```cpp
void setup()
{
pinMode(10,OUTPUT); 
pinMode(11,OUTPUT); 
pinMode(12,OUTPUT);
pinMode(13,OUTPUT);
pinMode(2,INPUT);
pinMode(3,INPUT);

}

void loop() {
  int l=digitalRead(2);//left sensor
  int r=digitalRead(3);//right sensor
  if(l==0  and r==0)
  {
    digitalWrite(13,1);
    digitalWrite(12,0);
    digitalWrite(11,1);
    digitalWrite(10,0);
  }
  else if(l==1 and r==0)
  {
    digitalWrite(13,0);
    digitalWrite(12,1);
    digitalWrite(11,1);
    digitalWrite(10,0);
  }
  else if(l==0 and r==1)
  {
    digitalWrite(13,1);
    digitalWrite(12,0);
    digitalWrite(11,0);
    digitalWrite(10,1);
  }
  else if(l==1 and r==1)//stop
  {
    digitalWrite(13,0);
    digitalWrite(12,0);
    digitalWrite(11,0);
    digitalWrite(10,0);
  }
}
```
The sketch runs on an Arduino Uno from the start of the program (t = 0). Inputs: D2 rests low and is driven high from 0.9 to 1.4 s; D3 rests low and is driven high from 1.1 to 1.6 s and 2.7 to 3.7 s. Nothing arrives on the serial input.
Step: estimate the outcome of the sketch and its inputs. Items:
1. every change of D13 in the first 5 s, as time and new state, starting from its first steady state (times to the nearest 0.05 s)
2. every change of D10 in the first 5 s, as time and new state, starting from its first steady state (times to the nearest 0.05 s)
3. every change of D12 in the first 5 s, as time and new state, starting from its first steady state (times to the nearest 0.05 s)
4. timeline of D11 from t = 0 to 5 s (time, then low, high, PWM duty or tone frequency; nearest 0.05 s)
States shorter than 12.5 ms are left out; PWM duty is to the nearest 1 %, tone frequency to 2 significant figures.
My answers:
0 s high; 0.9 s low; 1.4 s high
0 s low; 1.4 s high; 1.6 s low; 2.7 s high; 3.7 s low
0 s low; 0.9 s high; 1.1 s low
0 s high; 1.1 s low; 1.6 s high; 2.7 s low; 3.7 s high
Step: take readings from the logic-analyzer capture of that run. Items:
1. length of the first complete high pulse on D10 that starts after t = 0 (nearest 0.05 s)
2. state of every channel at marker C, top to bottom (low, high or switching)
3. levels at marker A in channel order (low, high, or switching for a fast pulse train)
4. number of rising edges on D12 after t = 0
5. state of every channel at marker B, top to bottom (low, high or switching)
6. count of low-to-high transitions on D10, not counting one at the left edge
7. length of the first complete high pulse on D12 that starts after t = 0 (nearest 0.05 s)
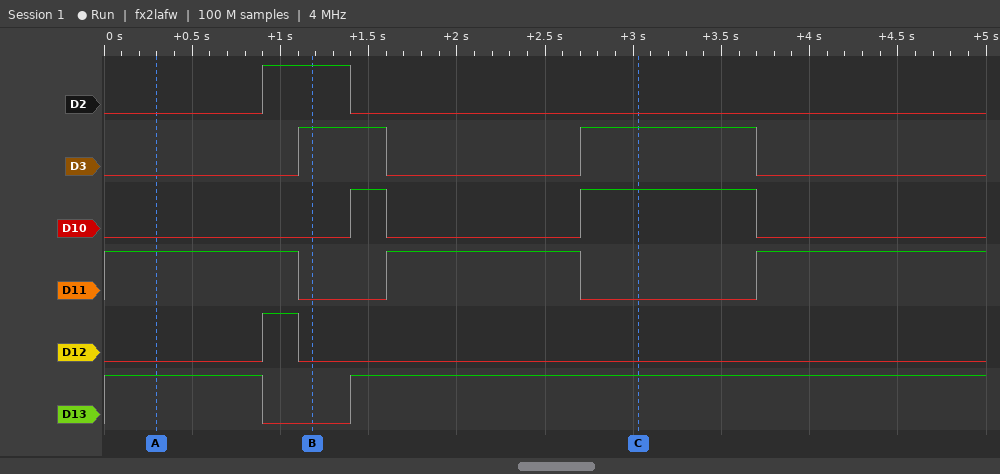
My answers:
0.20 s
D2 low, D3 high, D10 high, D11 low, D12 low, D13 high
D2 low, D3 low, D10 low, D11 high, D12 low, D13 high
1
D2 high, D3 high, D10 low, D11 low, D12 low, D13 low
2
0.20 s
